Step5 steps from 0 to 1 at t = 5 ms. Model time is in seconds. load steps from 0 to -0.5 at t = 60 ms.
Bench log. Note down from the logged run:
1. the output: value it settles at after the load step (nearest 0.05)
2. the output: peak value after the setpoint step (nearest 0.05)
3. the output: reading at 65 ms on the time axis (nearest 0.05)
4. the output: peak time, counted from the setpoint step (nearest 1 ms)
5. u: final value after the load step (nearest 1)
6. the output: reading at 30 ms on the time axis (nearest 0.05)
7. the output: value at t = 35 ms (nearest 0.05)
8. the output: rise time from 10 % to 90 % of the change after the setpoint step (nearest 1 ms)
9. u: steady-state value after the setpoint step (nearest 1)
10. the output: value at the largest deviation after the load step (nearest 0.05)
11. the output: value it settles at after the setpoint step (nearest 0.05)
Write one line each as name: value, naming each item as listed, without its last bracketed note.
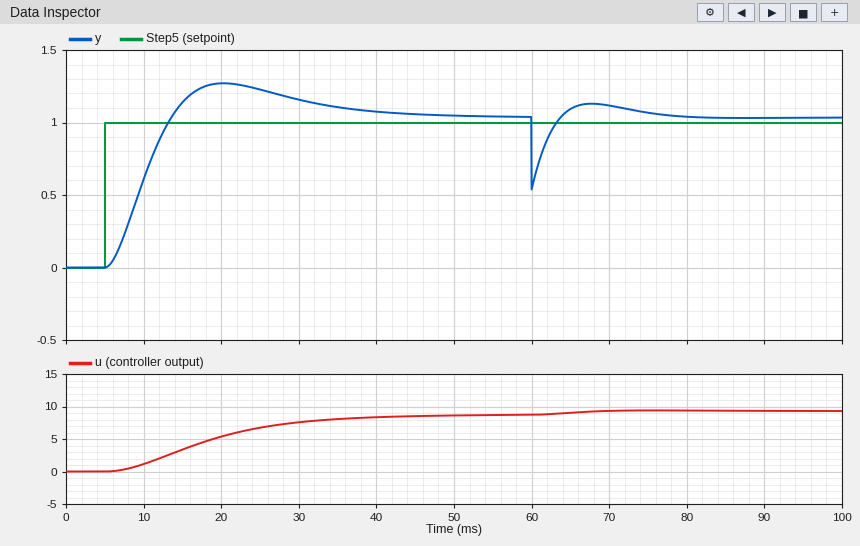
the output: value it settles at after the load step: 1.05
the output: peak value after the setpoint step: 1.25
the output: reading at 65 ms on the time axis: 1.10
the output: peak time, counted from the setpoint step: 15 ms
u: final value after the load step: 9
the output: reading at 30 ms on the time axis: 1.15
the output: value at t = 35 ms: 1.10
the output: rise time from 10 % to 90 % of the change after the setpoint step: 6 ms
u: steady-state value after the setpoint step: 9
the output: value at the largest deviation after the load step: 0.55
the output: value it settles at after the setpoint step: 1.05
